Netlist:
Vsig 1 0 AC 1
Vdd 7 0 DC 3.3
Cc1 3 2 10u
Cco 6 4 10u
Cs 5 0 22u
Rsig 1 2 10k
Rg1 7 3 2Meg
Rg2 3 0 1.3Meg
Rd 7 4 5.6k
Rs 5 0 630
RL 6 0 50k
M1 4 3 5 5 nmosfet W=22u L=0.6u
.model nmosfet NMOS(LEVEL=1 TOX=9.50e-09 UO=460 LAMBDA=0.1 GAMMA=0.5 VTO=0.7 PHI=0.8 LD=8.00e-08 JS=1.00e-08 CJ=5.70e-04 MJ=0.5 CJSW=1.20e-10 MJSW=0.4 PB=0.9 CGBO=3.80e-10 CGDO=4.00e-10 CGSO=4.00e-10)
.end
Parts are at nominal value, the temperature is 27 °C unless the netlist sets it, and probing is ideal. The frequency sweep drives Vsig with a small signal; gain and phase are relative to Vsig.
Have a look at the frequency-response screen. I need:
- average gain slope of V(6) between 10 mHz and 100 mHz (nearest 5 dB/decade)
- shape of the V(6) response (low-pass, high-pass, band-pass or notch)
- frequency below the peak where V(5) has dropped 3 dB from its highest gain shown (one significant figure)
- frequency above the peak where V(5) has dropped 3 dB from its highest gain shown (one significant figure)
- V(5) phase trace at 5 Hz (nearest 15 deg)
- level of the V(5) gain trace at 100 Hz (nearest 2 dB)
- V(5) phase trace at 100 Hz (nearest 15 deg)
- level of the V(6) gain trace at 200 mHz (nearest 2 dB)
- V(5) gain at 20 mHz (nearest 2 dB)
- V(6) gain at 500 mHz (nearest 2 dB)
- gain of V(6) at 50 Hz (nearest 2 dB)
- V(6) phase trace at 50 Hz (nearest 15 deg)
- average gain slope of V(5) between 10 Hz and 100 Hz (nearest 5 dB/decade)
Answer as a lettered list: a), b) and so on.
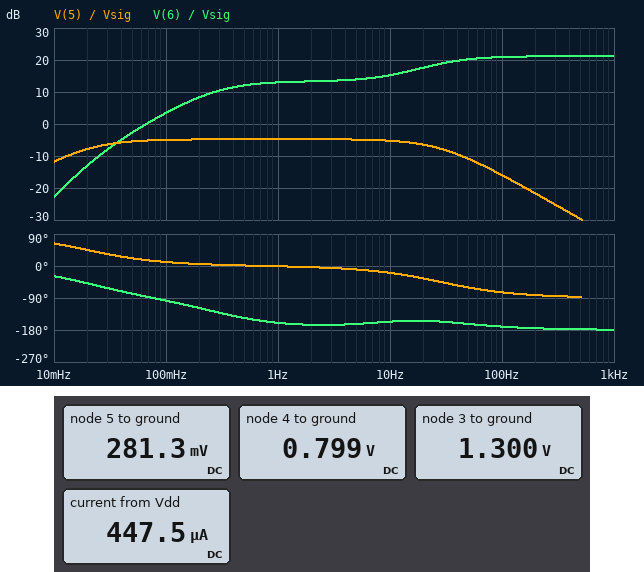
a) 25 dB/decade
b) high-pass
c) 20 mHz
d) 30 Hz
e) -15 deg
f) -16 dB
g) -75 deg
h) 8 dB
i) -8 dB
j) 12 dB
k) 20 dB
l) -165 deg
m) -10 dB/decade
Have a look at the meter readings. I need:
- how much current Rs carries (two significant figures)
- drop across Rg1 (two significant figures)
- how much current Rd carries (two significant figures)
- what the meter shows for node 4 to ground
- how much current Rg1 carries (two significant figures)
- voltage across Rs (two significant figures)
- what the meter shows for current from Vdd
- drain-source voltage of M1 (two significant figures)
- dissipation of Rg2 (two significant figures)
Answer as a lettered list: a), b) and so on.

a) 450 µA
b) 2.0 V
c) 450 µA
d) 0.799 V
e) 1.0 µA
f) 280 mV
g) 447.5 µA
h) 520 mV
i) 1.3 µW
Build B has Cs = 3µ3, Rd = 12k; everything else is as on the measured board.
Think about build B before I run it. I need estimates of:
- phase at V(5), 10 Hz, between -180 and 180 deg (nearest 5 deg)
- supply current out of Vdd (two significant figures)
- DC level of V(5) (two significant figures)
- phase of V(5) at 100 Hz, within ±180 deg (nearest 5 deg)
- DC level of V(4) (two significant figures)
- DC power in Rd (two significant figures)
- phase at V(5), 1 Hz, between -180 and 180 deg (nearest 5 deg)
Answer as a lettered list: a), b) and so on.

a) -5 deg
b) 260 µA
c) 160 mV
d) -50 deg
e) 240 mV
f) 780 µW
g) 5 deg
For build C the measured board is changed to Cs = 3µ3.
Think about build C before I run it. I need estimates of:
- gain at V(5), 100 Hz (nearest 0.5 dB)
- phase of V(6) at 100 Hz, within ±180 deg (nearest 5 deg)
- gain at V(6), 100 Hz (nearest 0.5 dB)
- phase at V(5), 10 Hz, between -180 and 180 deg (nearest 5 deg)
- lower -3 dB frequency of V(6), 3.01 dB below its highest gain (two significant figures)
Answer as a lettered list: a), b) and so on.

a) -6.0 dB
b) -155 deg
c) 16.5 dB
d) -5 deg
e) 160 Hz
